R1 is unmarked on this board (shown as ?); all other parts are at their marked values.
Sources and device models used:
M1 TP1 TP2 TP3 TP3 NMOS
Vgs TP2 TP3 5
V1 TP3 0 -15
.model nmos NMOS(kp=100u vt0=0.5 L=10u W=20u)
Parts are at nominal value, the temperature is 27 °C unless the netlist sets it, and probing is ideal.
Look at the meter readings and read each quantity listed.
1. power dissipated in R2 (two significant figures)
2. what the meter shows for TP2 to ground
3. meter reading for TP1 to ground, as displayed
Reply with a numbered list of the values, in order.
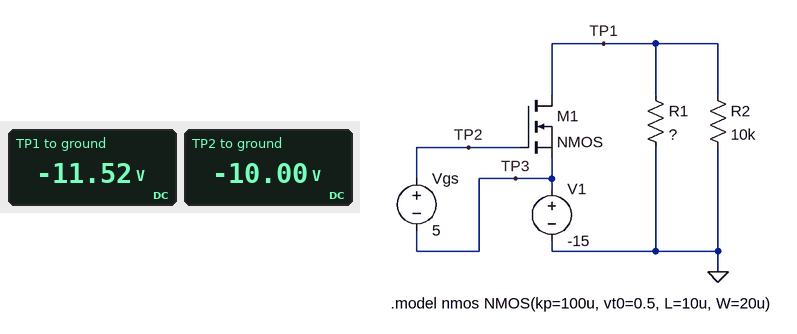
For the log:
1. 13 mW
2. -10.00 V
3. -11.52 V
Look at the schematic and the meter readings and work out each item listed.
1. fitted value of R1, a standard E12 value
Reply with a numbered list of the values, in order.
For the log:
1. 15 kΩ
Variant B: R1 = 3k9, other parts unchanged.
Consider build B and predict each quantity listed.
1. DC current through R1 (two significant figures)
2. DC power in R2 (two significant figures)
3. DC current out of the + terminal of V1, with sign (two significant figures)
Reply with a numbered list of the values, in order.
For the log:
1. 1.5 mA
2. 3.2 mW
3. -2.0 mA
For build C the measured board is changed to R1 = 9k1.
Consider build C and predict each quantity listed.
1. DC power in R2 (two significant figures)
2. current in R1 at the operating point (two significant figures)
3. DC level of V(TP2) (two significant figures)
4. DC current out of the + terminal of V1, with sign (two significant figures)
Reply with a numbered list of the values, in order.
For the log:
1. 9.3 mW
2. 1.1 mA
3. -10 V
4. -2.0 mA
